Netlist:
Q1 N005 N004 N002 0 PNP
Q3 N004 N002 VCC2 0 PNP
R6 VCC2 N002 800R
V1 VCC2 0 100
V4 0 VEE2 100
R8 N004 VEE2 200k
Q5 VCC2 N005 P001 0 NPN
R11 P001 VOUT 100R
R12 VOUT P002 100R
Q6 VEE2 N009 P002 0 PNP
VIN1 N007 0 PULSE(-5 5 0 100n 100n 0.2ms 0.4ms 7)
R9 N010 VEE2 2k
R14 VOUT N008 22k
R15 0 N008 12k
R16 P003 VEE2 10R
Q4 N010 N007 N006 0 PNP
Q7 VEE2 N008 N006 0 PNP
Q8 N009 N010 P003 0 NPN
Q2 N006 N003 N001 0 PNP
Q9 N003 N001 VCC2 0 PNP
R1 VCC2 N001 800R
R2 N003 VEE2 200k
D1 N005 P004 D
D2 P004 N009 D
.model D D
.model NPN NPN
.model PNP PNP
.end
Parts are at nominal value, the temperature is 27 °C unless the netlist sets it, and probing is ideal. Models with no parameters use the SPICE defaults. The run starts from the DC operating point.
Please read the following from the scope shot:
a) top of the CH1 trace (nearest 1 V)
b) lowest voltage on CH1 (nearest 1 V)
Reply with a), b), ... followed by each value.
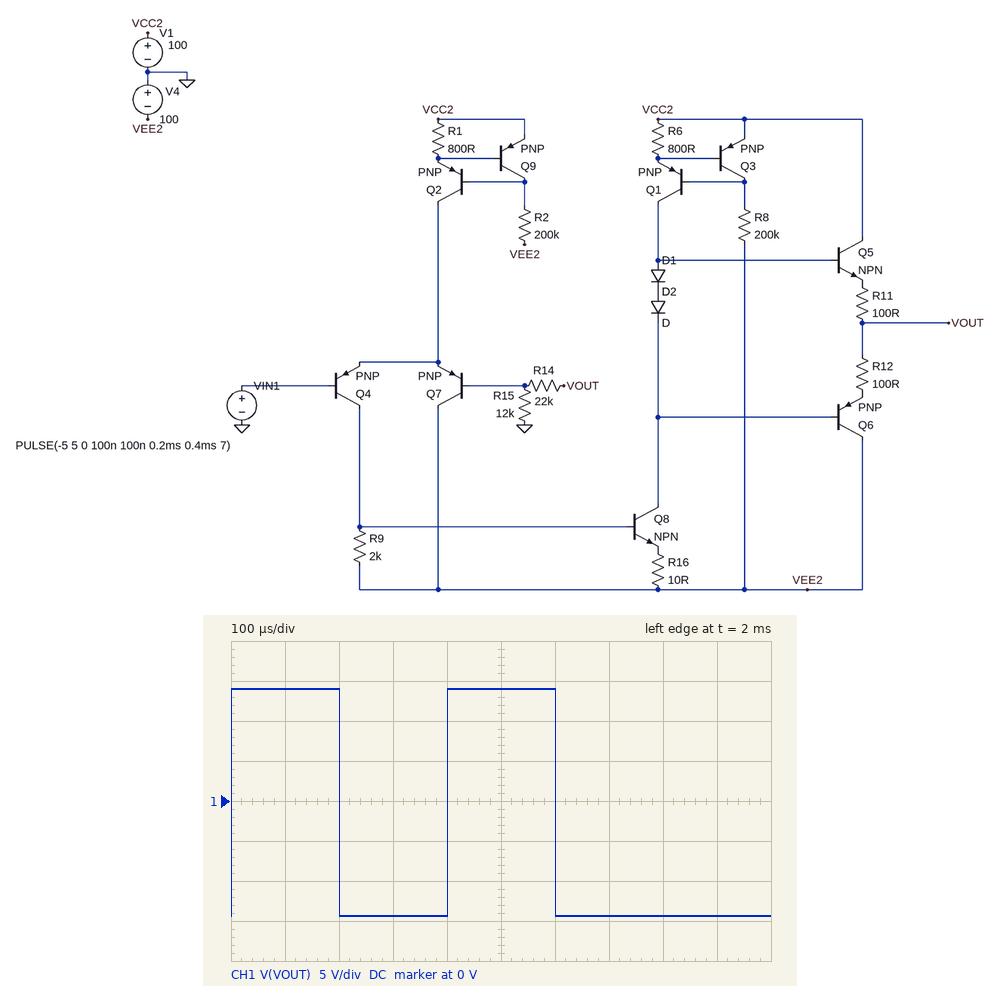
a) 14 V
b) -14 V
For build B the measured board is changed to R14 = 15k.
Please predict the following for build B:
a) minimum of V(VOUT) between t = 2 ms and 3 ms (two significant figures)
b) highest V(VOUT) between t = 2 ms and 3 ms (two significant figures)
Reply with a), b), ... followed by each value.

a) -11 V
b) 11 V
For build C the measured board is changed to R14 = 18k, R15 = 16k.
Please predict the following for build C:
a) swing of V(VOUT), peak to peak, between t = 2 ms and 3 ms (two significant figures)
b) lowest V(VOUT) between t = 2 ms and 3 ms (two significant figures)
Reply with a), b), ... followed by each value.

a) 21 V
b) -11 V
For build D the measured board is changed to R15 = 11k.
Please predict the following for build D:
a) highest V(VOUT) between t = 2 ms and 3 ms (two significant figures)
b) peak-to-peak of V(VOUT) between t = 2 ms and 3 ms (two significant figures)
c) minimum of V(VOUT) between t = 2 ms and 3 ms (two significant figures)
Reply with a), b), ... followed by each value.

a) 15 V
b) 30 V
c) -15 V
